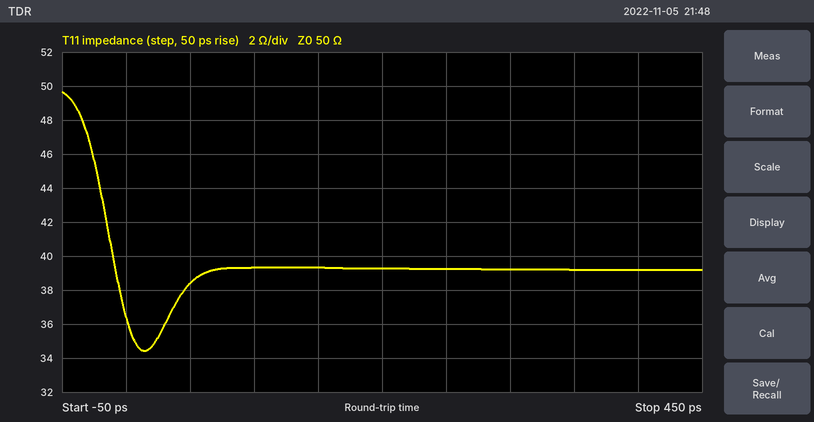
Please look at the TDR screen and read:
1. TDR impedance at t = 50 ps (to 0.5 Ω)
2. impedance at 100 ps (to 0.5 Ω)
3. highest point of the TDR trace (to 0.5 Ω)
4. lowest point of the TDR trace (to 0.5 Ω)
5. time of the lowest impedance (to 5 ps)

38.5 Ω
39.5 Ω
49.5 Ω
34.5 Ω
15 ps
